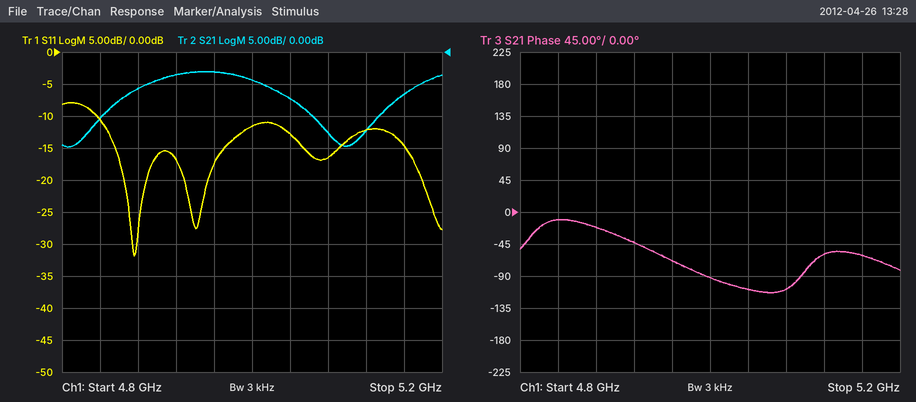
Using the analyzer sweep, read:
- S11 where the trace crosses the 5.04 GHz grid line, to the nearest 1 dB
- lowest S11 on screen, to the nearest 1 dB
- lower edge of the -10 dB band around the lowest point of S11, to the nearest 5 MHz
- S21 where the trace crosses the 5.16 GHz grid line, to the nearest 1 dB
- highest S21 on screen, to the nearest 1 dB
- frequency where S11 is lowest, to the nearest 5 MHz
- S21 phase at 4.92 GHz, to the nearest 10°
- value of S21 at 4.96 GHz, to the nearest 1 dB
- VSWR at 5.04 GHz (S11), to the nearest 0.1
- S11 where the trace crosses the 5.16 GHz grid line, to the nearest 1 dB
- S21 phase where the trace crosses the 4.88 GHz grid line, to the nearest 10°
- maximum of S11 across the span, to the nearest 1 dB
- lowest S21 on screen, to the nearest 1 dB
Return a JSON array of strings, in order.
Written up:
["-13 dB", "-32 dB", "4.835 GHz", "-7 dB", "-3 dB", "4.875 GHz", "-40°", "-3 dB", "1.6", "-15 dB", "-20°", "-8 dB", "-15 dB"]
